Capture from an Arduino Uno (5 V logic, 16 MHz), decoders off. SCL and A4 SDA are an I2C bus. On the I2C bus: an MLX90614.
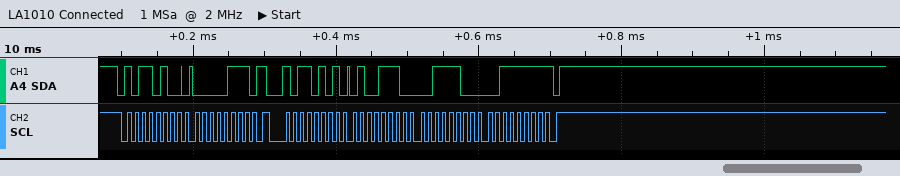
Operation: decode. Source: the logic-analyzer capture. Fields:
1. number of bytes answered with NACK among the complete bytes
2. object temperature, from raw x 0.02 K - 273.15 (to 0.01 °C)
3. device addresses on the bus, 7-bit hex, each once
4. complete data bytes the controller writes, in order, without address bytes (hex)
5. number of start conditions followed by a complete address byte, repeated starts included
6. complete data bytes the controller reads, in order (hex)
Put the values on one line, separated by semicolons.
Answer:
1; 35.61 °C; 0x5A; 07; 2; 4E 3C 3F
